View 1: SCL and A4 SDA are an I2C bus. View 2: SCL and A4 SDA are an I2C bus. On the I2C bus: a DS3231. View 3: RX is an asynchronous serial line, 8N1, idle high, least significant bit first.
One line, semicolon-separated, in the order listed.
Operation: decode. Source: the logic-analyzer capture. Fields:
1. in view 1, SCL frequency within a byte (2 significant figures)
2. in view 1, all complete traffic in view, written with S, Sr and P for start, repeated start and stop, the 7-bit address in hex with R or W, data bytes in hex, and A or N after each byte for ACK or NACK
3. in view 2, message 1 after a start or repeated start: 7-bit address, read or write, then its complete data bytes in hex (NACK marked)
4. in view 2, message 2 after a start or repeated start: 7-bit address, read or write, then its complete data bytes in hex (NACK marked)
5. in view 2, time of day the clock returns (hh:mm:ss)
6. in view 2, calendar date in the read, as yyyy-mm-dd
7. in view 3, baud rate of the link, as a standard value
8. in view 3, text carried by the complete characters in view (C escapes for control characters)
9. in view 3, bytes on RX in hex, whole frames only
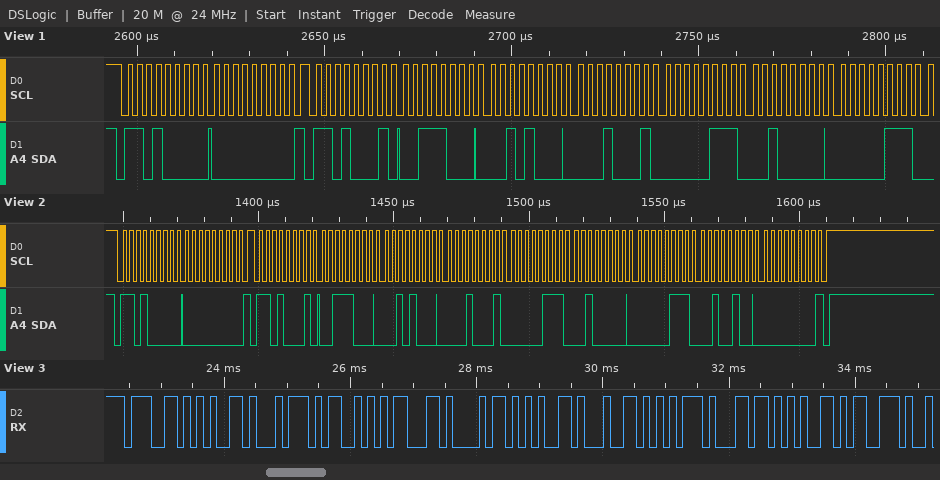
400 kHz; S 68W A 00 A Sr 68R A 38 A 28 A 11 A 07 A 20 A 07 A; 0x68 write: 00; 0x68 read: 38 28 11 07 20 07 24 00 NACK; 11:28:38; 2024-07-20; 9600 baud; "getSchedules"; 67 65 74 53 63 68 65 64 75 6C 65 73
